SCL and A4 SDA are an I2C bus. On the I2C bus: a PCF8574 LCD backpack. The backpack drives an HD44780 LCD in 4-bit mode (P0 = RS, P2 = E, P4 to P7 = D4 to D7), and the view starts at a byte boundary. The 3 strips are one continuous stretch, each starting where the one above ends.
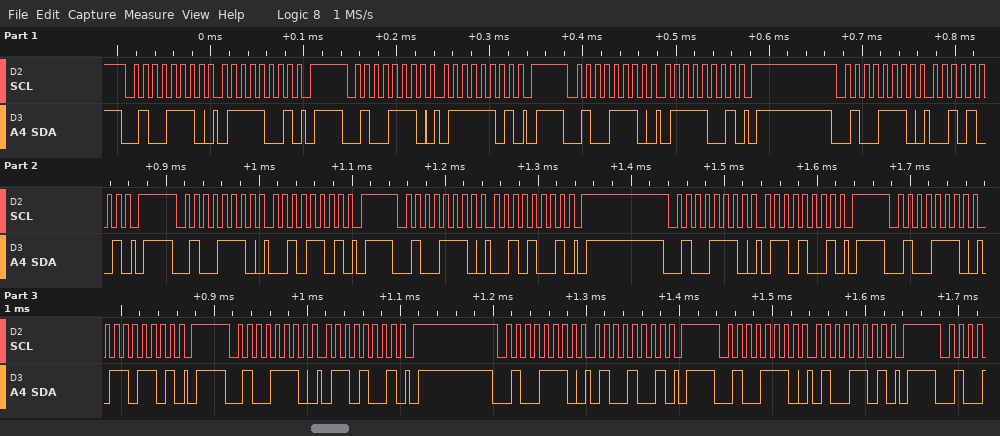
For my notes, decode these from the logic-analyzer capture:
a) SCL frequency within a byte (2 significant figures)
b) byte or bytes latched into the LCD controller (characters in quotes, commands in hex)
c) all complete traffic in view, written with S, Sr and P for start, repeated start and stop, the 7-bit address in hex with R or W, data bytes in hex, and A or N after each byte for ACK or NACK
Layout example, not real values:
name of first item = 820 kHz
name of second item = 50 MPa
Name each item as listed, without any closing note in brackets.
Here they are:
SCL frequency within a byte = 100 kHz
byte or bytes latched into the LCD controller = 'r'
all complete traffic in view, written with S, Sr and P for start, repeated start and stop, the 7-bit address in hex with R or W, data bytes in hex, and A or N after each byte for ACK or NACK = S 27W A 79 A P S 27W A 7D A P S 27W A 79 A P S 27W A 29 A P S 27W A 2D A P S 27W A 29 A P S 27W A 69 A P S 27W A 6D A P S 27W A 69 A P S 27W A 49 A P S 27W A 4D A P
